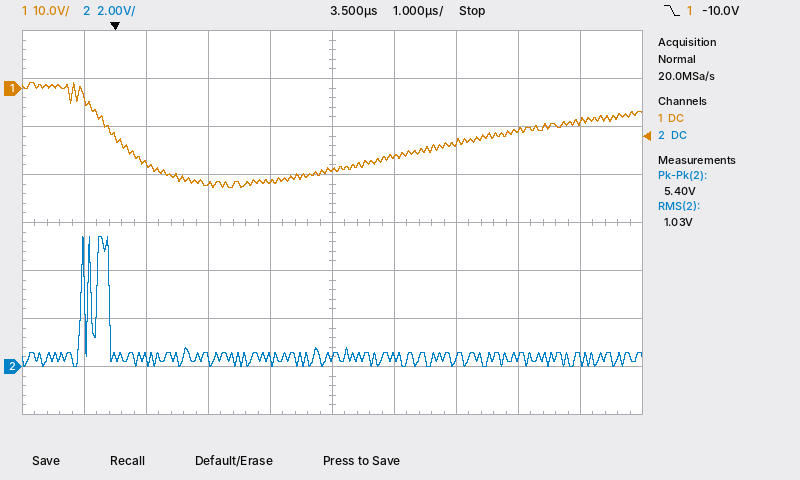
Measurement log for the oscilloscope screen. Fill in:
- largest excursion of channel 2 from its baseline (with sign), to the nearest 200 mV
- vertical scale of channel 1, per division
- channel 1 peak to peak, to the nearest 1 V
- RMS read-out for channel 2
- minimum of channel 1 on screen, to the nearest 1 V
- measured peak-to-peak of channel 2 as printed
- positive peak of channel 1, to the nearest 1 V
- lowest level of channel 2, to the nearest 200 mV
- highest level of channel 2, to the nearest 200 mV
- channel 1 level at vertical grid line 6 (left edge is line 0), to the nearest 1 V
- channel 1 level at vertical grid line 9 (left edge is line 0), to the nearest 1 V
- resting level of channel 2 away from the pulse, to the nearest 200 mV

+5.0 V
10 V
22 V
1.03 V
-21 V
5.40 V
1 V
0.0 V
5.4 V
-14 V
-7 V
400 mV
